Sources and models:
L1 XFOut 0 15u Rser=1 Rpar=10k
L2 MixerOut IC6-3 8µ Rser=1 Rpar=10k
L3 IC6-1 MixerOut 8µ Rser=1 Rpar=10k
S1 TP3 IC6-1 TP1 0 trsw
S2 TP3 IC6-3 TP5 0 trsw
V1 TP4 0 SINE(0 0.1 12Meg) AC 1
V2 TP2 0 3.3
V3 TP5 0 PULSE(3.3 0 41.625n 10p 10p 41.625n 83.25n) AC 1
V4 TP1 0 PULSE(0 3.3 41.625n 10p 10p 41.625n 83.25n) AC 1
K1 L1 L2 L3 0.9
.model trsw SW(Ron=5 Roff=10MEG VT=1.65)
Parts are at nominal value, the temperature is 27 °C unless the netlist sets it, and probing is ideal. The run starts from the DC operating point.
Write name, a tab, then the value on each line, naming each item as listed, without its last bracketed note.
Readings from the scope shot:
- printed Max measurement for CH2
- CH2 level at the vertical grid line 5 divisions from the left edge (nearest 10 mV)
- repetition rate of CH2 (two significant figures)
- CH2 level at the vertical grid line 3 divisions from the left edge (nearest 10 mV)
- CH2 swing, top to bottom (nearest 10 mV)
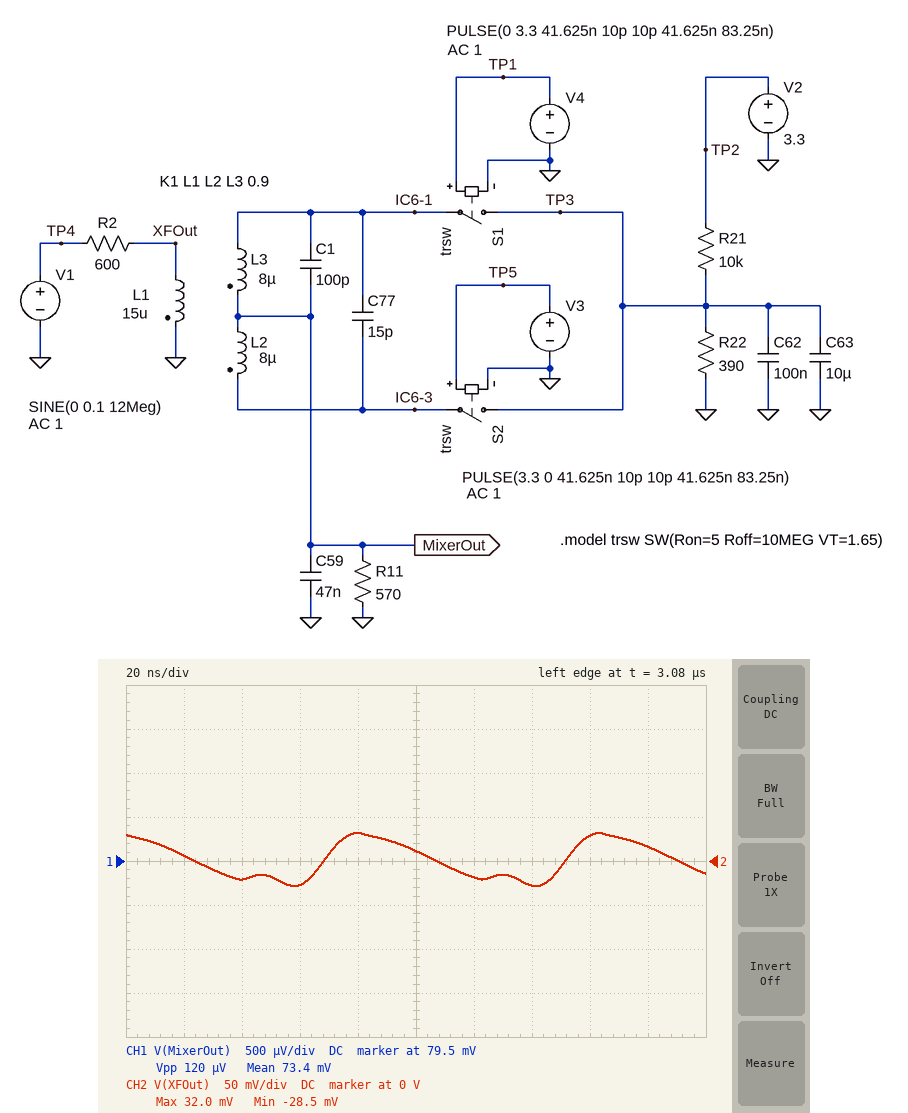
printed Max measurement for CH2	32.0 mV
CH2 level at the vertical grid line 5 divisions from the left edge	10 mV
repetition rate of CH2	12 MHz
CH2 level at the vertical grid line 3 divisions from the left edge	-30 mV
CH2 swing, top to bottom	60 mV
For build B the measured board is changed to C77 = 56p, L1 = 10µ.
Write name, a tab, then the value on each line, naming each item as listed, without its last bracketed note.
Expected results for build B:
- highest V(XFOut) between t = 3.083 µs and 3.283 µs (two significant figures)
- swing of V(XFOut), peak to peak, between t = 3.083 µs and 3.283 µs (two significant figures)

highest V(XFOut) between t = 3.083 µs and 3.283 µs	16 mV
swing of V(XFOut), peak to peak, between t = 3.083 µs and 3.283 µs	34 mV
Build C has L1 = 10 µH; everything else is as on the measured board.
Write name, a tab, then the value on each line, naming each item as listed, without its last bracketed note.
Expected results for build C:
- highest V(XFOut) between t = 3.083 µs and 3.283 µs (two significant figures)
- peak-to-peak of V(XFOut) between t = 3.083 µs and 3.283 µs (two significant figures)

highest V(XFOut) between t = 3.083 µs and 3.283 µs	25 mV
peak-to-peak of V(XFOut) between t = 3.083 µs and 3.283 µs	43 mV
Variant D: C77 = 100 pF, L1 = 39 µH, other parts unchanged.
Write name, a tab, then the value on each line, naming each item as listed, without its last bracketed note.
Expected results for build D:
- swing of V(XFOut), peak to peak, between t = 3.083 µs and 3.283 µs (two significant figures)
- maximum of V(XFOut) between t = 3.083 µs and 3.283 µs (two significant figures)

swing of V(XFOut), peak to peak, between t = 3.083 µs and 3.283 µs	100 mV
maximum of V(XFOut) between t = 3.083 µs and 3.283 µs	51 mV
